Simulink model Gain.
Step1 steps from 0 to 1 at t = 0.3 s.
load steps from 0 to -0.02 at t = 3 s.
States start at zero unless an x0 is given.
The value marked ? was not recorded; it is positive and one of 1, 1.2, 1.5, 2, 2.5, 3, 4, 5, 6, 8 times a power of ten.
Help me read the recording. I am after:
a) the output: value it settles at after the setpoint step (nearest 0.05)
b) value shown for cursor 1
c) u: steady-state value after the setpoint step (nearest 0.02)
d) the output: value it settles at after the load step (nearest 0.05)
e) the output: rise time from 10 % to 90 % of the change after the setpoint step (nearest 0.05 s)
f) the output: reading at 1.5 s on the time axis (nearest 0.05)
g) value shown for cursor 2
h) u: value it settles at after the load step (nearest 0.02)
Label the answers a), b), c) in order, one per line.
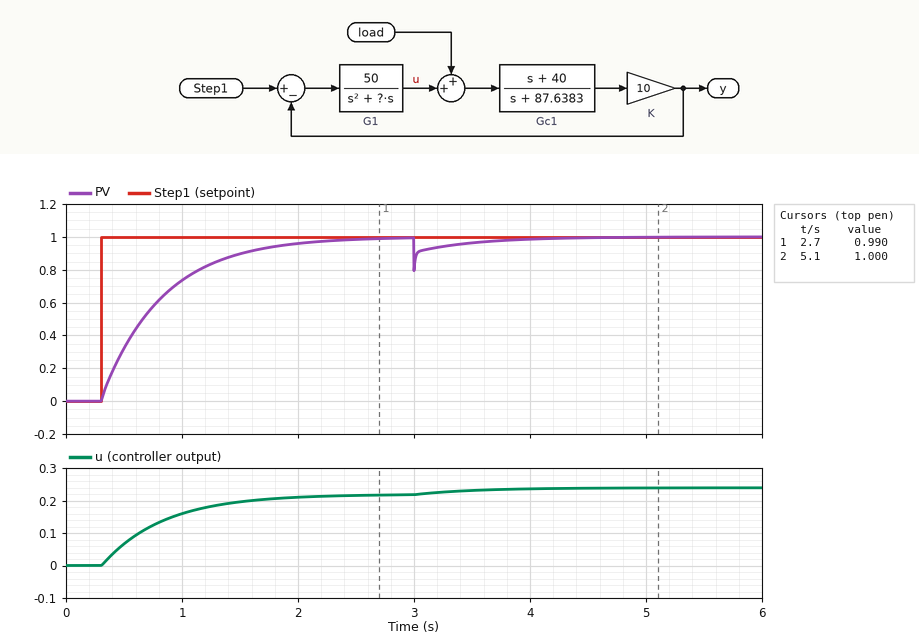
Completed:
a) 1.00
b) 0.990
c) 0.22
d) 1.00
e) 1.15 s
f) 0.90
g) 1.000
h) 0.24
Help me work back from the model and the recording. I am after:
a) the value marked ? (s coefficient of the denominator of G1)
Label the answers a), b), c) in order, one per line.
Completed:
a) 120
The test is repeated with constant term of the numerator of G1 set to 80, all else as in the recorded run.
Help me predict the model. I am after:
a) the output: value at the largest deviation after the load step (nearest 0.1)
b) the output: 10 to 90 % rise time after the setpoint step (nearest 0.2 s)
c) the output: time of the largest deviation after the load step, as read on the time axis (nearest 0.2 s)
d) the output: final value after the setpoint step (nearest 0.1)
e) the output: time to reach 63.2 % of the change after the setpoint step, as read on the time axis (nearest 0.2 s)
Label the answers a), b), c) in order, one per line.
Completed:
a) 0.8
b) 0.8 s
c) 3.0 s
d) 1.0
e) 0.6 s
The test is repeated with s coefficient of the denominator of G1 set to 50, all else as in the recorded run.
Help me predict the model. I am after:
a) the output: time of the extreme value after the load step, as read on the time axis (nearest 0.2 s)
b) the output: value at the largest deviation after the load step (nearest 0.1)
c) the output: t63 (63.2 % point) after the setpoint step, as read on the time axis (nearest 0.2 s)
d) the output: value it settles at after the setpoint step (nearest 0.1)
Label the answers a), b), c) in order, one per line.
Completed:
a) 3.0 s
b) 0.8
c) 0.6 s
d) 1.0
